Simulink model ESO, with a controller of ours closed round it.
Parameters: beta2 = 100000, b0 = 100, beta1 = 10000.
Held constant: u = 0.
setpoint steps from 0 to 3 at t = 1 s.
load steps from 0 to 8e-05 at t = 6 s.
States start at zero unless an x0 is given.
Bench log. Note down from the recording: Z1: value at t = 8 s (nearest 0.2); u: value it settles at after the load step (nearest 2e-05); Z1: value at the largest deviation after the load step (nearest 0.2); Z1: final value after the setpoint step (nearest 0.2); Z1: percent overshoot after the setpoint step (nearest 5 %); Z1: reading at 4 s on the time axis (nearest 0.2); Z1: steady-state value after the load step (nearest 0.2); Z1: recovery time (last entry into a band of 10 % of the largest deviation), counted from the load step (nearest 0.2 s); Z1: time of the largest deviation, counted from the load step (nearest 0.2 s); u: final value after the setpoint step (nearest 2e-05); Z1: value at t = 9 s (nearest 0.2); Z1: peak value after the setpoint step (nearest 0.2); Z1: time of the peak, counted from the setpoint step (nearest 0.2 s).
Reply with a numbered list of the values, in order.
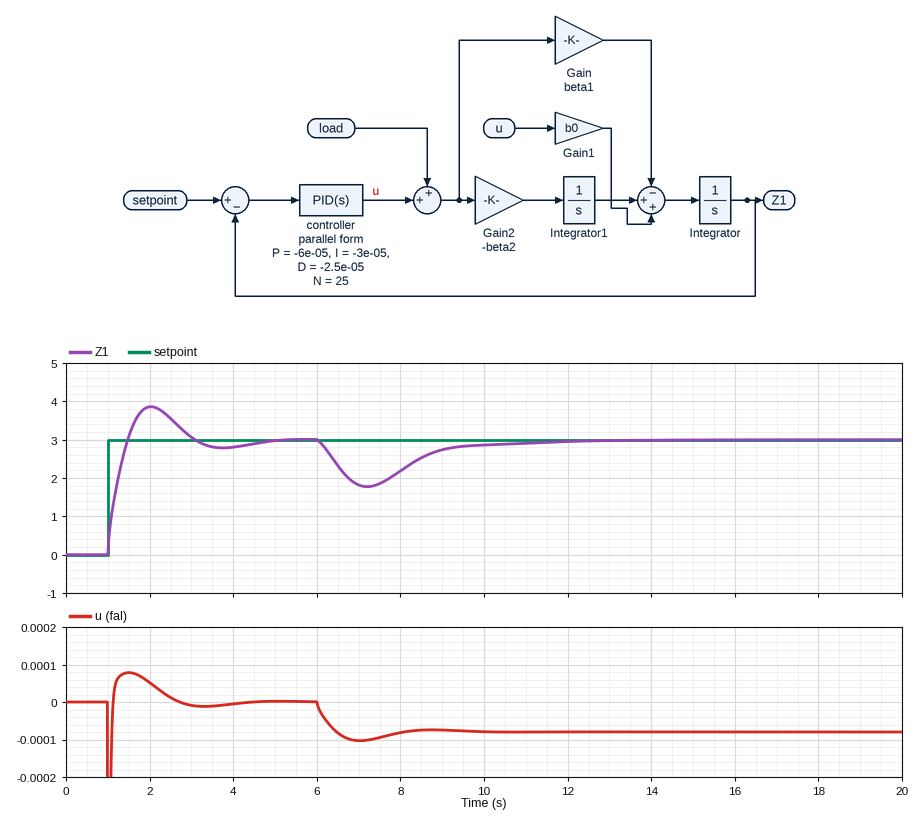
1. 2.2
2. -0.00008
3. 1.8
4. 3.0
5. 30 %
6. 2.8
7. 3.0
8. 4.4 s
9. 1.2 s
10. 0.00000
11. 2.8
12. 3.8
13. 1.0 s
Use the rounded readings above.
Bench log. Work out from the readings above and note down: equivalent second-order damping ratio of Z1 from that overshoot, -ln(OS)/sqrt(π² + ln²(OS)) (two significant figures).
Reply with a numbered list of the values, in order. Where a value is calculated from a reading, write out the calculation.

1. ln(0.3) = -1.204; 1.204 / sqrt(9.870 + 1.450) = 0.36
